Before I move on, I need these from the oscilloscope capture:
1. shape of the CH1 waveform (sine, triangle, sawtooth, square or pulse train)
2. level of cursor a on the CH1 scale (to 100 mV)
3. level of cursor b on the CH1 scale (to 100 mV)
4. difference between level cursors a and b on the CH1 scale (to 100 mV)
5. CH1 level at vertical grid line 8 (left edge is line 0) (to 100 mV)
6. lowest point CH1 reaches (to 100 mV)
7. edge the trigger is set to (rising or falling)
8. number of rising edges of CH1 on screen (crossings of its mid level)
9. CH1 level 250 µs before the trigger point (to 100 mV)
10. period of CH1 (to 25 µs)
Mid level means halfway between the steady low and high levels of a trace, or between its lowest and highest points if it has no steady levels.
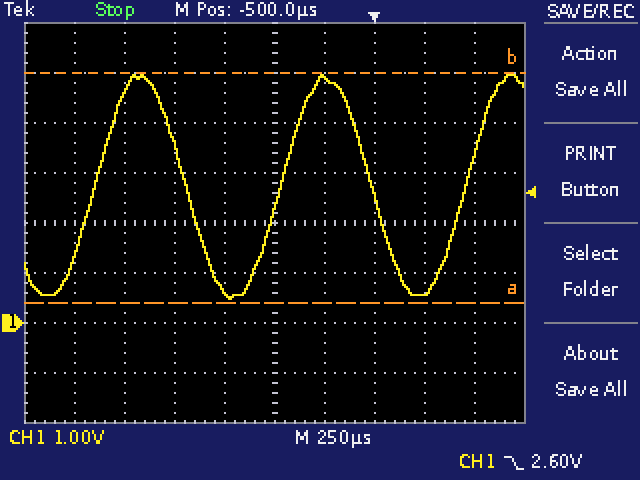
sine
400 mV
5.0 V
4.6 V
600 mV
500 mV
falling
3
4.9 V
925 µs
